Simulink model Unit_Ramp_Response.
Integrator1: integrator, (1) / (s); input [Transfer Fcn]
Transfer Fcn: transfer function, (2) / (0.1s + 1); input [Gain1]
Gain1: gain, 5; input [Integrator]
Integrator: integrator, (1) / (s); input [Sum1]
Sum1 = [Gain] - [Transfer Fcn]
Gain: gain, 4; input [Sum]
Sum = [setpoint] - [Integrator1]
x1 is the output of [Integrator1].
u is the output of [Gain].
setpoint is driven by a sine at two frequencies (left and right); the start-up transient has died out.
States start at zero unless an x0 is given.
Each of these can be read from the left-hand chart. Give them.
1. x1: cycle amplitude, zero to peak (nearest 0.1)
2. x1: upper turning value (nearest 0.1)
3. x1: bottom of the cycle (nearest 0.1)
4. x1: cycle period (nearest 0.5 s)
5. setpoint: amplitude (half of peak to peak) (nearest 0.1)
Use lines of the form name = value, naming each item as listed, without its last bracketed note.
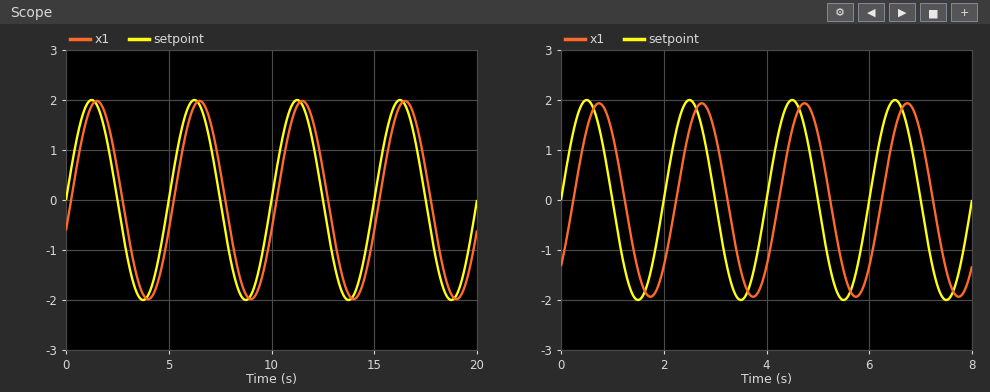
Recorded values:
x1: cycle amplitude, zero to peak = 2.0
x1: upper turning value = 2.0
x1: bottom of the cycle = -2.0
x1: cycle period = 5.0 s
setpoint: amplitude (half of peak to peak) = 2.0
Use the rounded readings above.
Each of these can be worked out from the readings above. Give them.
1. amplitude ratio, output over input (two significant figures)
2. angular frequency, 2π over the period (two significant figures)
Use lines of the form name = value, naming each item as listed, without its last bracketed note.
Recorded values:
amplitude ratio, output over input = 1.0
angular frequency, 2π over the period = 1.3 rad/s
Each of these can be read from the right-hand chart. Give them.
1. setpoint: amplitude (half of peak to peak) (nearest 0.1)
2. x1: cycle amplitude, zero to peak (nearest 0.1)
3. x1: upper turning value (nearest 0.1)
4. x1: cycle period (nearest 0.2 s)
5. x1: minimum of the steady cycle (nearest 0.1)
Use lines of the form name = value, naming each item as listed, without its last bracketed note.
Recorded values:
setpoint: amplitude (half of peak to peak) = 2.0
x1: cycle amplitude, zero to peak = 1.9
x1: upper turning value = 1.9
x1: cycle period = 2.0 s
x1: minimum of the steady cycle = -1.9
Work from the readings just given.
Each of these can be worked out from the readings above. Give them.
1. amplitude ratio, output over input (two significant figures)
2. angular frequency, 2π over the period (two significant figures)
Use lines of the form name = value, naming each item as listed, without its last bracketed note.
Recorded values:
amplitude ratio, output over input = 0.95
angular frequency, 2π over the period = 3.1 rad/s
